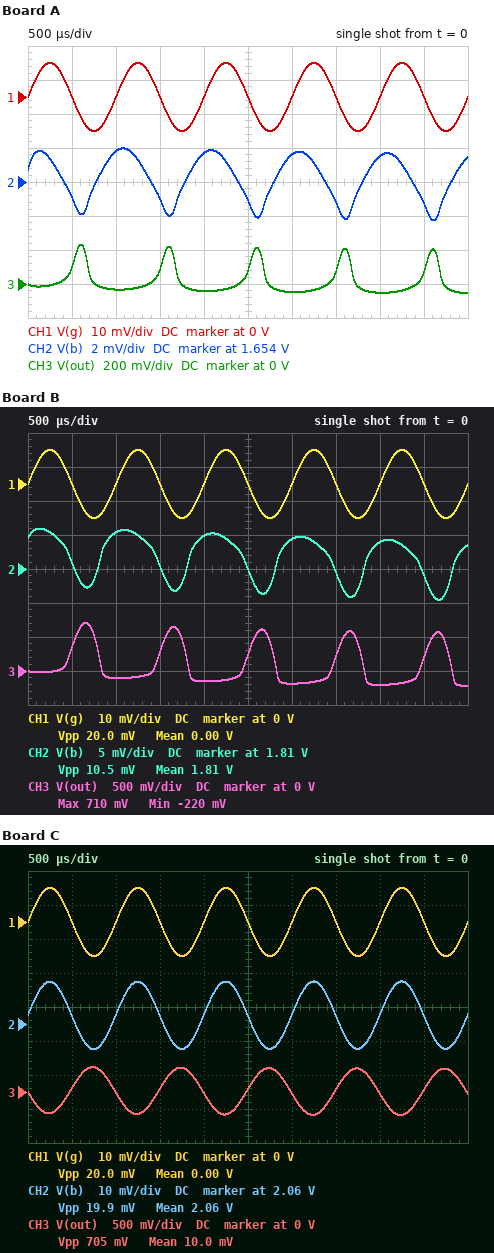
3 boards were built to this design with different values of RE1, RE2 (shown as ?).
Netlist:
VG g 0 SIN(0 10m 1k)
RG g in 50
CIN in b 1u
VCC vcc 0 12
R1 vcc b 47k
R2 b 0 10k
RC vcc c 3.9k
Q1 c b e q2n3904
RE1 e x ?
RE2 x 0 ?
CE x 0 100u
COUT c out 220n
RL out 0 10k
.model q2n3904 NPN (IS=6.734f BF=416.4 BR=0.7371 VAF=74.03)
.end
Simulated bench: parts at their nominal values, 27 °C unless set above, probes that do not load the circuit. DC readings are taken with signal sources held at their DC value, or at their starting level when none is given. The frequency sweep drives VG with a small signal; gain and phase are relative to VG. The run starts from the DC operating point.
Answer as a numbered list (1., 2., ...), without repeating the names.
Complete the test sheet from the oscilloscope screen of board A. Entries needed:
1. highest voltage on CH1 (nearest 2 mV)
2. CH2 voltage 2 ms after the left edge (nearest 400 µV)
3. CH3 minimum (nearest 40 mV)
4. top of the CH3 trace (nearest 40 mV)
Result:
1. 10 mV
2. 1.6556 V
3. -40 mV
4. 240 mV
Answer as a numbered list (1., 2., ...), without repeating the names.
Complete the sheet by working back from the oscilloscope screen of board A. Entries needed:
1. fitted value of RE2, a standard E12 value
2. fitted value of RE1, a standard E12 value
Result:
1. 330 Ω
2. 6.8 Ω
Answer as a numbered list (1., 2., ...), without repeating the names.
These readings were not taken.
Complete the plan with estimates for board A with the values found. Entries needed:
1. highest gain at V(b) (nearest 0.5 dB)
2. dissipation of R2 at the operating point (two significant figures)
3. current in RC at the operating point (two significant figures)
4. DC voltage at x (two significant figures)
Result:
1. -9.5 dB
2. 270 µW
3. 2.8 mA
4. 940 mV
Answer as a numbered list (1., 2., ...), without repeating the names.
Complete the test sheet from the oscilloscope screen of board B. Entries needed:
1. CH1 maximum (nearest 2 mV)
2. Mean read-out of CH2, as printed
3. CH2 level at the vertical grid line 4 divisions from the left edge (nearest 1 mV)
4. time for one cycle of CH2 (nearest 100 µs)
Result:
1. 10 mV
2. 1.81 V
3. 1.815 V
4. 1.0 ms
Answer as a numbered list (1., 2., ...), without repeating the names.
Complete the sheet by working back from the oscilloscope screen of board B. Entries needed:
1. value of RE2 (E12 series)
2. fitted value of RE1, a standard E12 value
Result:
1. 390 Ω
2. 12 Ω
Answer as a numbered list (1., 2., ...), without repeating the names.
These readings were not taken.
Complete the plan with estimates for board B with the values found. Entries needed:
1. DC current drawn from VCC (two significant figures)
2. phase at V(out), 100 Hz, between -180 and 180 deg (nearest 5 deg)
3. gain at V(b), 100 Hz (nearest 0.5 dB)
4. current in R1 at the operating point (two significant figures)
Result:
1. 3.0 mA
2. -55 deg
3. -32.0 dB
4. 220 µA
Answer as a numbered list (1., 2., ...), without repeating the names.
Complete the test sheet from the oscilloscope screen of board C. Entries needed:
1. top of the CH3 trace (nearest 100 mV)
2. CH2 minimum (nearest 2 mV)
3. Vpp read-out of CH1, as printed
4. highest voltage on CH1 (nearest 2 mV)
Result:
1. 400 mV
2. 2.052 V
3. 20.0 mV
4. 10 mV
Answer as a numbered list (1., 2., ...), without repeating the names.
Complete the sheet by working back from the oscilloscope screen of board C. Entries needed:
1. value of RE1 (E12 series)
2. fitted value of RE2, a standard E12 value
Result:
1. 68 Ω
2. 560 Ω
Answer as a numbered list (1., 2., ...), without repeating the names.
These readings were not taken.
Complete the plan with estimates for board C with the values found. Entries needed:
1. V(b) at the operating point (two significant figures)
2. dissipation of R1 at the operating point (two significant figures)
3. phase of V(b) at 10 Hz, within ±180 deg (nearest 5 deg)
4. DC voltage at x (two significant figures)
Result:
1. 2.1 V
2. 2.1 mW
3. 60 deg
4. 1.2 V
